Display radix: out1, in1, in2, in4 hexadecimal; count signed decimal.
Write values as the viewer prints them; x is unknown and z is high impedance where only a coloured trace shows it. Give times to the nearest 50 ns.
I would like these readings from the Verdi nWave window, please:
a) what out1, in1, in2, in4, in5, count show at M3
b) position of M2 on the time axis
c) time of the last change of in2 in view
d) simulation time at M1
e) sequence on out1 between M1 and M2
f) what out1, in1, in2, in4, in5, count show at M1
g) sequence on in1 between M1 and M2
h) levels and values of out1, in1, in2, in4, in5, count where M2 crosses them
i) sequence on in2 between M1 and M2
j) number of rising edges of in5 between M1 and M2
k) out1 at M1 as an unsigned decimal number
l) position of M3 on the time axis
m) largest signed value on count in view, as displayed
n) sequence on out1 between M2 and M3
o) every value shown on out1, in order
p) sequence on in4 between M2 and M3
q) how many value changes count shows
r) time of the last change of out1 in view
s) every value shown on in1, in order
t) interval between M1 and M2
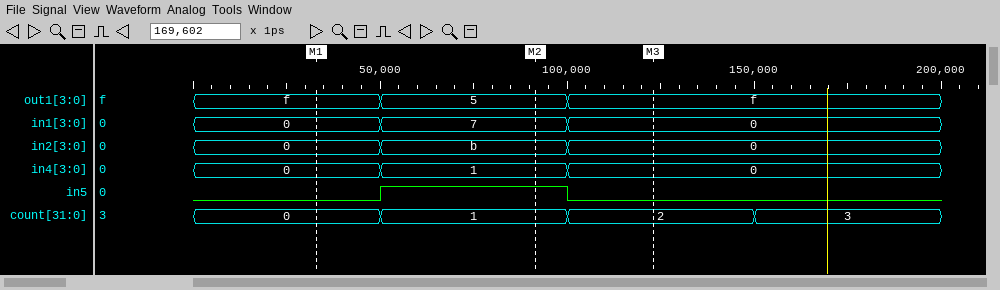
out1=f, in1=0, in2=0, in4=0, in5=0, count=2
100 ns
100 ns
50 ns
f, 5
out1=f, in1=0, in2=0, in4=0, in5=0, count=0
0, 7
out1=5, in1=7, in2=b, in4=1, in5=1, count=1
0, b
1
15
100 ns
3
5, f
f, 5, f
1, 0
3
100 ns
0, 7, 0
50 ns
